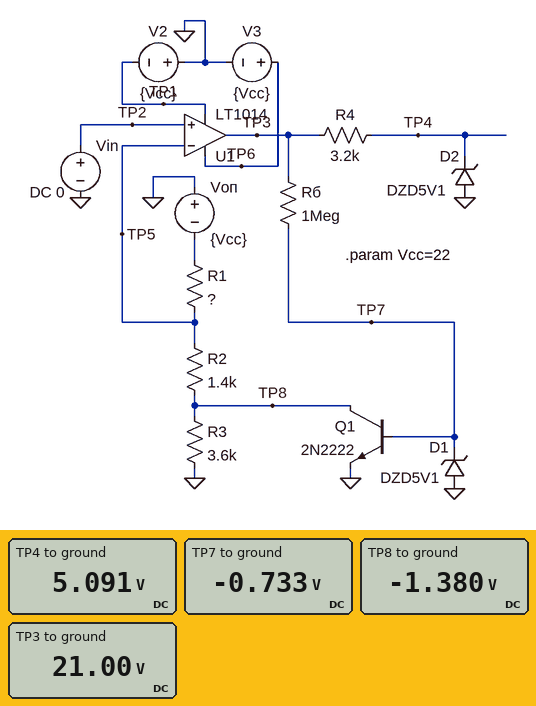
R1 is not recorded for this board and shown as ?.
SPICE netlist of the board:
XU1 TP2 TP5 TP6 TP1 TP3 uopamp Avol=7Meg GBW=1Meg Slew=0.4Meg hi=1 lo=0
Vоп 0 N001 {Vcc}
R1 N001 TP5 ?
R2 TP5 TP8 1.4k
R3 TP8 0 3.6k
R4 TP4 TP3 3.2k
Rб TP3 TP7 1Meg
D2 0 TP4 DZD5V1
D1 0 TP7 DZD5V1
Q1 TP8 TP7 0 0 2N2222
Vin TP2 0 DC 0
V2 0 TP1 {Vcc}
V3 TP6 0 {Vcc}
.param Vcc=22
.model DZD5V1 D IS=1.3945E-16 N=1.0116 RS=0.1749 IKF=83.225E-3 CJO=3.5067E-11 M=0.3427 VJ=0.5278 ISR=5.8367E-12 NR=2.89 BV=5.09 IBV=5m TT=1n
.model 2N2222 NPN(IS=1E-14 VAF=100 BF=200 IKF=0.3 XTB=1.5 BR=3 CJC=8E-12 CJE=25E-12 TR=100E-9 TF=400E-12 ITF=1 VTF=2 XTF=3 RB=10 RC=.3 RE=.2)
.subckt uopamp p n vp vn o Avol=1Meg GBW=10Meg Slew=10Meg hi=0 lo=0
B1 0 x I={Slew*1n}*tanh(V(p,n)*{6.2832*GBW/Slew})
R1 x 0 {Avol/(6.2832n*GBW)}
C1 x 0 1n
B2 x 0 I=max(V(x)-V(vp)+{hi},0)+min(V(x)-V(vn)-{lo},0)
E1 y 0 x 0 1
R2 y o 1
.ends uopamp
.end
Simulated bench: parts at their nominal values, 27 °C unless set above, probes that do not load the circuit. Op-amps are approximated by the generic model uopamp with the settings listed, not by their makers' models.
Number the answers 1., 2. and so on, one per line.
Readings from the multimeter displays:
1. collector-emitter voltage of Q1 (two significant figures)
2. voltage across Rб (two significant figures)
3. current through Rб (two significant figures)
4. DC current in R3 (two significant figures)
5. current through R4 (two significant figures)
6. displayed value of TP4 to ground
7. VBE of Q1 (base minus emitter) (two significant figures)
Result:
1. -1.4 V
2. 22 V
3. 22 µA
4. 380 µA
5. 5.0 mA
6. 5.091 V
7. -730 mV
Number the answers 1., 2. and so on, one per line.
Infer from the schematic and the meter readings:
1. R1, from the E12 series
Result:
1. 15 kΩ
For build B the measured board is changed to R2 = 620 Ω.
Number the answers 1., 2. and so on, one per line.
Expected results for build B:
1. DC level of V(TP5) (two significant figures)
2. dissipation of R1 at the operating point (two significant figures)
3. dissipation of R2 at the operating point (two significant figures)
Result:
1. -2.2 V
2. 26 mW
3. 1.1 mW
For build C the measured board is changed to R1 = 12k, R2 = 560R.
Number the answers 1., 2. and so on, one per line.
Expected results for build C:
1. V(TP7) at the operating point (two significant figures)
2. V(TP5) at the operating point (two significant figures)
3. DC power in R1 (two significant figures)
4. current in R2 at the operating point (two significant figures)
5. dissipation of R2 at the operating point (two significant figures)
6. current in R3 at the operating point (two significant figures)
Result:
1. -740 mV
2. -2.3 V
3. 32 mW
4. 1.6 mA
5. 1.5 mW
6. 390 µA
